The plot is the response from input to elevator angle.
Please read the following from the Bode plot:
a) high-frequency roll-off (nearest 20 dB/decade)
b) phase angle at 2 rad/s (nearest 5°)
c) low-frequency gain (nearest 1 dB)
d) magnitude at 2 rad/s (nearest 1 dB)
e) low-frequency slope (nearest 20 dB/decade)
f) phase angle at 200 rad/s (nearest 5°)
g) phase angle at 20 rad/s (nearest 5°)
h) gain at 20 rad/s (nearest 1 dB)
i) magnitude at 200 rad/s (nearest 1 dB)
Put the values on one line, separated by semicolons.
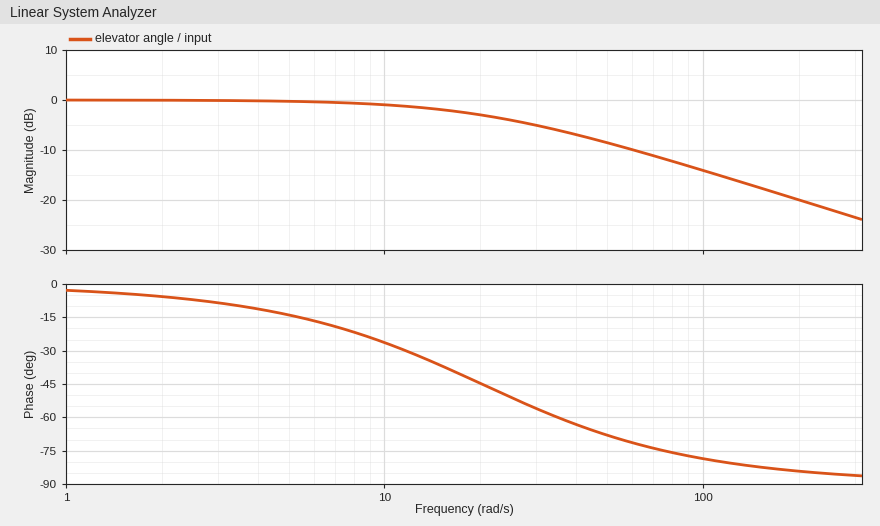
-20 dB/decade; -5°; 0 dB; 0 dB; 0 dB/decade; -85°; -45°; -3 dB; -20 dB
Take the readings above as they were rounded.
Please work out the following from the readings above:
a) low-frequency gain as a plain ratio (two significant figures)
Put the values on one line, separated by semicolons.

1.0
